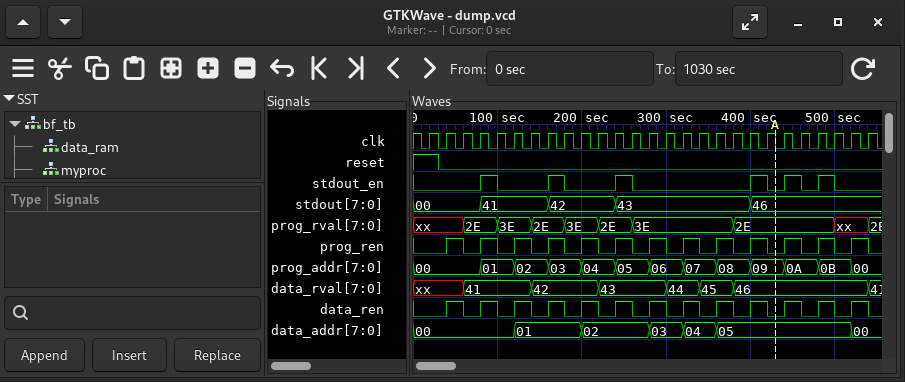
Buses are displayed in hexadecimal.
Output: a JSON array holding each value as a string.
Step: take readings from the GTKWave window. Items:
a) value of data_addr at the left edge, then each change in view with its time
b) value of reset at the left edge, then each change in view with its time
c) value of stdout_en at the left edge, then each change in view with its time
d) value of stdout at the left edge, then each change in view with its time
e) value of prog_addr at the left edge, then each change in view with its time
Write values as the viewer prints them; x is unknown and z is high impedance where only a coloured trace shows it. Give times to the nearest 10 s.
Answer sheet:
["00, 01 at 120 s, 02 at 200 s, 03 at 280 s, 04 at 320 s, 05 at 360 s, 00 at 520 s", "1, 0 at 30 s", "0, 1 at 80 s, 0 at 100 s, 1 at 160 s, 0 at 180 s, 1 at 240 s, 0 at 260 s, 1 at 400 s, 0 at 420 s, 1 at 440 s, 0 at 460 s, 1 at 480 s, 0 at 500 s", "00, 41 at 80 s, 42 at 160 s, 43 at 240 s, 46 at 400 s", "00, 01 at 80 s, 02 at 120 s, 03 at 160 s, 04 at 200 s, 05 at 240 s, 06 at 280 s, 07 at 320 s, 08 at 360 s, 09 at 400 s, 0A at 440 s, 0B at 480 s, 00 at 520 s"]
